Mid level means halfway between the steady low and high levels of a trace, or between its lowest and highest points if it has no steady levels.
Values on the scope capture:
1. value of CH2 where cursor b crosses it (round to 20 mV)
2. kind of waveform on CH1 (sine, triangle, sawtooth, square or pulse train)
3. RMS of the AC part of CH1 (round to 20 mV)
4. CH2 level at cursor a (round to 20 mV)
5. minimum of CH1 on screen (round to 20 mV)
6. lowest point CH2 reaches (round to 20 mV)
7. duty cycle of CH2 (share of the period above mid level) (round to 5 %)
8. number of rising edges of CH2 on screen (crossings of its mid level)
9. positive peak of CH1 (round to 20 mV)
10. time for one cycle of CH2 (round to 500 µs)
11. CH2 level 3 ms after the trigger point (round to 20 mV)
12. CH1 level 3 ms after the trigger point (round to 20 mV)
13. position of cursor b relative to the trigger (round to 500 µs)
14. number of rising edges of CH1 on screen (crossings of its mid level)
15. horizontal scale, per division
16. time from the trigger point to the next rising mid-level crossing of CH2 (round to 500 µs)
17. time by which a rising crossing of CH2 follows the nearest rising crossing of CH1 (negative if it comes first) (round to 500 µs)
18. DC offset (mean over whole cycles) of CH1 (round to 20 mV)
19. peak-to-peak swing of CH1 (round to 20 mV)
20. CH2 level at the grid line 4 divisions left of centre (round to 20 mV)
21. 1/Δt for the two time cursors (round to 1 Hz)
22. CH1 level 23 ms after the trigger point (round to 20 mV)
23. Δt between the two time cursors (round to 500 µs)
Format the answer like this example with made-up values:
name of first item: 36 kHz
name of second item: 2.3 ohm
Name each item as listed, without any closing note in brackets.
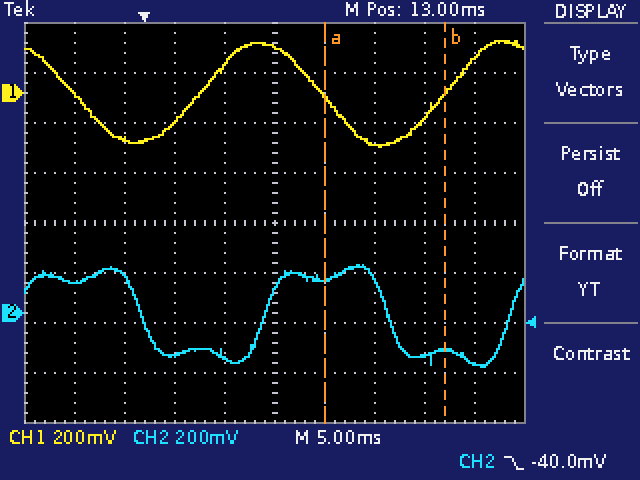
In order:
value of CH2 where cursor b crosses it: -140 mV
kind of waveform on CH1: sine
RMS of the AC part of CH1: 140 mV
CH2 level at cursor a: 140 mV
minimum of CH1 on screen: -220 mV
lowest point CH2 reaches: -220 mV
duty cycle of CH2 (share of the period above mid level): 50 %
number of rising edges of CH2 on screen: 2
positive peak of CH1: 200 mV
time for one cycle of CH2: 24.5 ms
CH2 level 3 ms after the trigger point: -160 mV
CH1 level 3 ms after the trigger point: -120 mV
position of cursor b relative to the trigger: +30.0 ms
number of rising edges of CH1 on screen: 2
horizontal scale, per division: 5 ms
time from the trigger point to the next rising mid-level crossing of CH2: 12.0 ms
time by which a rising crossing of CH2 follows the nearest rising crossing of CH1 (negative if it comes first): +6.5 ms
DC offset (mean over whole cycles) of CH1: 0 mV
peak-to-peak swing of CH1: 420 mV
CH2 level at the grid line 4 divisions left of centre: 120 mV
1/Δt for the two time cursors: 83 Hz
CH1 level 23 ms after the trigger point: -200 mV
Δt between the two time cursors: 12.0 ms
